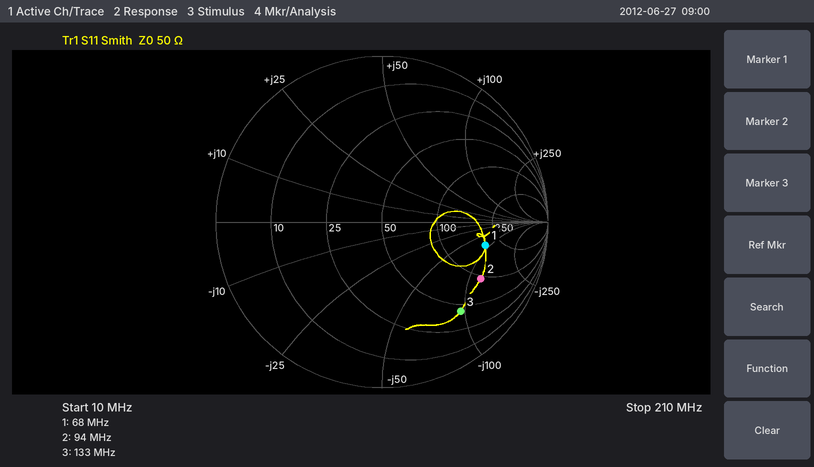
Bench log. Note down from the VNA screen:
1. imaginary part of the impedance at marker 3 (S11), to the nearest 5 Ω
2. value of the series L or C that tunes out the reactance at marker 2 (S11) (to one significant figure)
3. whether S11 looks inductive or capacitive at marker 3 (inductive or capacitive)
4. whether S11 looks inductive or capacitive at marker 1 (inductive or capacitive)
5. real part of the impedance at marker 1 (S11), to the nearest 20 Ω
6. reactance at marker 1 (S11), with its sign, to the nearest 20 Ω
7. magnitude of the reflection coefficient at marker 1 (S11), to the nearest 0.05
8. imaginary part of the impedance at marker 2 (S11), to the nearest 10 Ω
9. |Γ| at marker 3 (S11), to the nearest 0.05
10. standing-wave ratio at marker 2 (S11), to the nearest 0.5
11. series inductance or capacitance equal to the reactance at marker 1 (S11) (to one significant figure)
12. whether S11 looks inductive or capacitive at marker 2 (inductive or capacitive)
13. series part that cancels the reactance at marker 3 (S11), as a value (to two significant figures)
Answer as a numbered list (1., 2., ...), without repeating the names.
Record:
1. -95 Ω
2. 200 nH
3. capacitive
4. capacitive
5. 180 Ω
6. -80 Ω
7. 0.65
8. -120 Ω
9. 0.70
10. 5.5
11. 30 pF
12. capacitive
13. 110 nH
